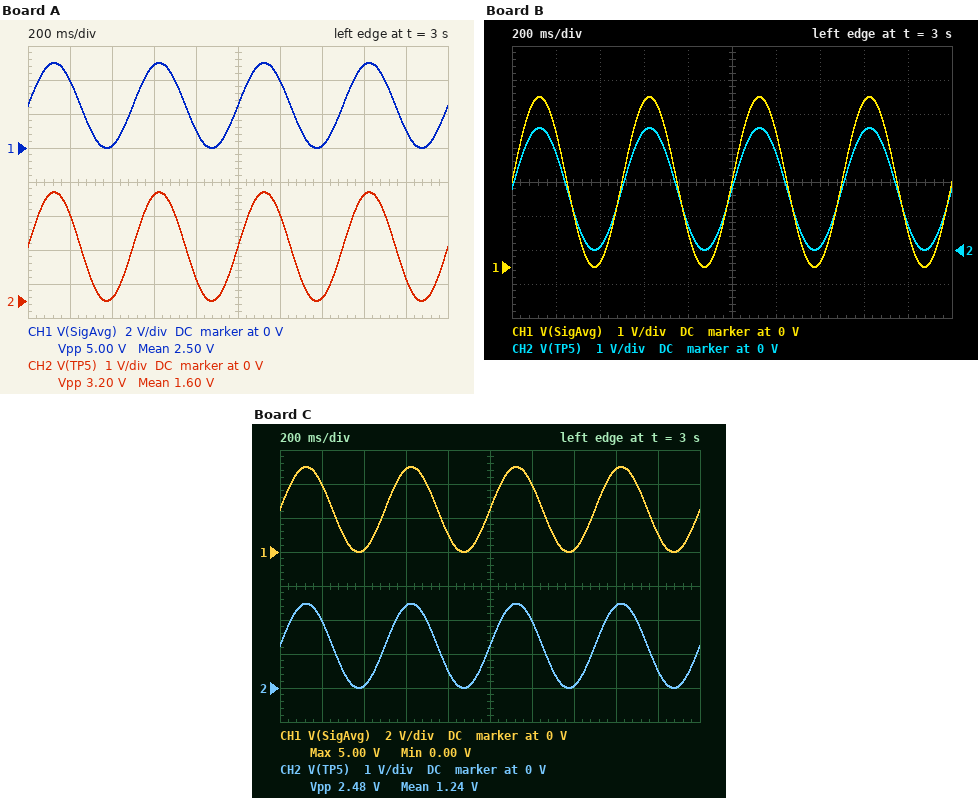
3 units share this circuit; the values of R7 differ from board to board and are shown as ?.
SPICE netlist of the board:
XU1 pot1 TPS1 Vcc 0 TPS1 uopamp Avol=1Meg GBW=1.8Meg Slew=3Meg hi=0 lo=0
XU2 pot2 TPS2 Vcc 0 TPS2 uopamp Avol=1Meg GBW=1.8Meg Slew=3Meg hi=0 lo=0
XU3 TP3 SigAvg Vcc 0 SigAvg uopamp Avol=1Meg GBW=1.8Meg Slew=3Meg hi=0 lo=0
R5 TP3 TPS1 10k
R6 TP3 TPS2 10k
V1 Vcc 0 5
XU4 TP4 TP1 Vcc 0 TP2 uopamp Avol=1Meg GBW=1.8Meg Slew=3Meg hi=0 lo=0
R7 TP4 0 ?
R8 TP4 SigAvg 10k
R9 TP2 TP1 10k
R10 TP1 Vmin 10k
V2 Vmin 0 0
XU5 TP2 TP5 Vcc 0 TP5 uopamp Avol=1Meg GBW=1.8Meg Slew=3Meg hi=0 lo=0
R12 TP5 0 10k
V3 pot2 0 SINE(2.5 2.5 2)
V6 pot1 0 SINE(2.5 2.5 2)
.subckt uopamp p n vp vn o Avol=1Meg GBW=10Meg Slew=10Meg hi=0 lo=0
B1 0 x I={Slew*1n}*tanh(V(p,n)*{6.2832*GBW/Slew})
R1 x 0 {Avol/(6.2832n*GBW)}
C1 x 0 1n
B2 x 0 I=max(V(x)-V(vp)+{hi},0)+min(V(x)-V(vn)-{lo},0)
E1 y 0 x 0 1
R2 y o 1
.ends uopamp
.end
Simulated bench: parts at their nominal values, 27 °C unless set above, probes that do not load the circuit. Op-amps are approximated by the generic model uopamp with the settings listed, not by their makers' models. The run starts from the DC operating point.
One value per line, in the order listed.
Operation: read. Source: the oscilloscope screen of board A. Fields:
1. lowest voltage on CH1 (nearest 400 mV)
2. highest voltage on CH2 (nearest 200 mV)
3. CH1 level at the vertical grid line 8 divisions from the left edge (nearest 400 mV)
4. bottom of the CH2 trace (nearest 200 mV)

0 V
3.2 V
4.8 V
0 V
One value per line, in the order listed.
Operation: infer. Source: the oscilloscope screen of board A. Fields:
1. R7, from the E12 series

4.7 kΩ
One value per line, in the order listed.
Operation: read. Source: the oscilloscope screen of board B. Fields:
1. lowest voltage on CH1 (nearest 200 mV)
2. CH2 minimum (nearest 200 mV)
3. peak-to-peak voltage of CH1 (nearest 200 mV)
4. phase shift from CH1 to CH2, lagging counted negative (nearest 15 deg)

0 V
0 V
5.0 V
0 deg
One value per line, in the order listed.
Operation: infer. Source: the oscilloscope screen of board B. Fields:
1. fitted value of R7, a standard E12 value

5.6 kΩ
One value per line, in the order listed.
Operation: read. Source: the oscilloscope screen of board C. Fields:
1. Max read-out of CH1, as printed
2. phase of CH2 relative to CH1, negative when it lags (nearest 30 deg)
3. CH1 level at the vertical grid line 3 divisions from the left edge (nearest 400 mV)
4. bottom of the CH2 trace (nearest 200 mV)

5.00 V
0 deg
4.8 V
0 V
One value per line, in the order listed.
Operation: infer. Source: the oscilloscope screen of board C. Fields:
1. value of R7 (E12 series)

3.3 kΩ
